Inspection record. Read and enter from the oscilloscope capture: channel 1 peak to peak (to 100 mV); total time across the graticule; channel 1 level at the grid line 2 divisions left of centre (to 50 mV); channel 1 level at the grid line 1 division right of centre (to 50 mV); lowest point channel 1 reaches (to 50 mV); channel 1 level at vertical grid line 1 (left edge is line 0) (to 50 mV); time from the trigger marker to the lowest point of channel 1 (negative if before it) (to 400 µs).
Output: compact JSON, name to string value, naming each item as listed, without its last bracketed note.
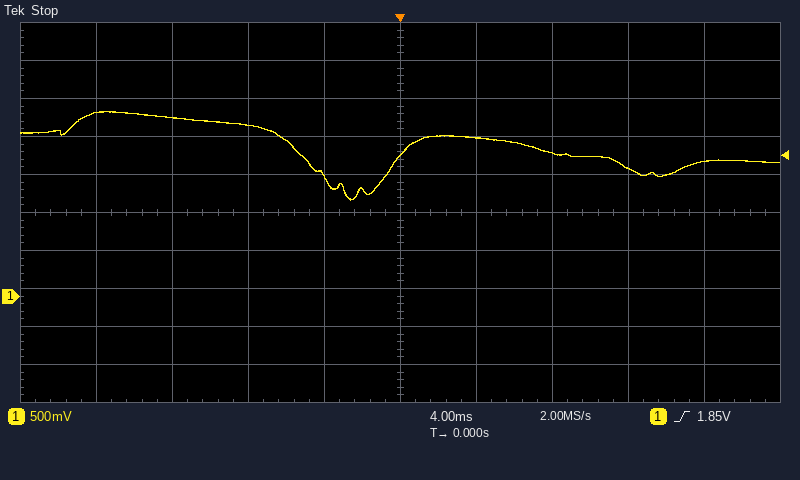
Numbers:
{"channel 1 peak to peak": "1.20 V", "total time across the graticule": "40 ms", "channel 1 level at the grid line 2 divisions left of centre": "2.25 V", "channel 1 level at the grid line 1 division right of centre": "2.10 V", "lowest point channel 1 reaches": "1.25 V", "channel 1 level at vertical grid line 1 (left edge is line 0)": "2.40 V", "time from the trigger marker to the lowest point of channel 1 (negative if before it)": "-2.4 ms"}
